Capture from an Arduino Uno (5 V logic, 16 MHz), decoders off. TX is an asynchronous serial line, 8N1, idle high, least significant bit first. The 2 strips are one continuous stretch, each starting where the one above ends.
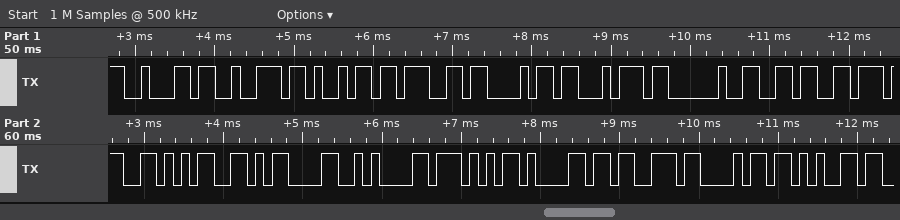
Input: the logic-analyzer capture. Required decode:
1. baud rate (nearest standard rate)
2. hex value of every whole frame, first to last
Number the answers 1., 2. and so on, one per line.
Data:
1. 9600 baud
2. 0x62 0x72 0x69 0x67 0x68 0x74 0x20 0x36 0x37 0x35 0x0D 0x0A 0x57 0x61 0x73 0x68 0x65
